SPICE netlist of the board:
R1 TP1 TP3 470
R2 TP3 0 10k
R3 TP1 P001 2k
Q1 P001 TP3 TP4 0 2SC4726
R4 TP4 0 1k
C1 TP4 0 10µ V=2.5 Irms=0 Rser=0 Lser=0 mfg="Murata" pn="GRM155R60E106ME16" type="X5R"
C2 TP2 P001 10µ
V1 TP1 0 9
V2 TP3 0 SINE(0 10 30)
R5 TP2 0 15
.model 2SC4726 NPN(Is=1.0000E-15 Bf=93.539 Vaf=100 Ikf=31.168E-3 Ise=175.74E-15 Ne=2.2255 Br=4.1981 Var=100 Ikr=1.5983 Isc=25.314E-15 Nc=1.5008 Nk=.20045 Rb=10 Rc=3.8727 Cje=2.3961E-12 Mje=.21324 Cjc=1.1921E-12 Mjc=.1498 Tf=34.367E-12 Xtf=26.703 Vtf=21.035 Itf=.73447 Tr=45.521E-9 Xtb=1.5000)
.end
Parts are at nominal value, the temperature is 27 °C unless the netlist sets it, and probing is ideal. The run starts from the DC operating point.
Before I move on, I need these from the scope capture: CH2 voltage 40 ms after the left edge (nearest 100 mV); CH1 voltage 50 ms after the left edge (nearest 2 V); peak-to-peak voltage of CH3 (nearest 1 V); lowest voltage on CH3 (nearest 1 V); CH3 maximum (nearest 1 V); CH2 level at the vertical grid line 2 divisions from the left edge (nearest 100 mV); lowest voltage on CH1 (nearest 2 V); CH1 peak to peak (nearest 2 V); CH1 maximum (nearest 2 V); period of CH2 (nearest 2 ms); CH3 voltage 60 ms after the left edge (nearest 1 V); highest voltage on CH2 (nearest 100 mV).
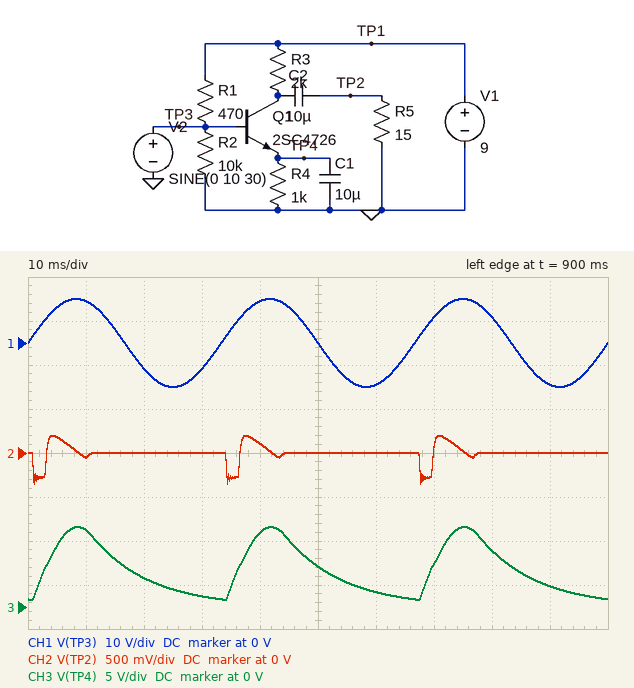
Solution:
100 mV
0 V
8 V
1 V
9 V
0 V
-10 V
20 V
10 V
34 ms
2 V
200 mV
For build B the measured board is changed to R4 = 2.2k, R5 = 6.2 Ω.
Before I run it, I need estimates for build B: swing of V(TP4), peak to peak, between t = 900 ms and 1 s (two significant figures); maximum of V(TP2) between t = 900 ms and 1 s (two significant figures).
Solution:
6.3 V
73 mV
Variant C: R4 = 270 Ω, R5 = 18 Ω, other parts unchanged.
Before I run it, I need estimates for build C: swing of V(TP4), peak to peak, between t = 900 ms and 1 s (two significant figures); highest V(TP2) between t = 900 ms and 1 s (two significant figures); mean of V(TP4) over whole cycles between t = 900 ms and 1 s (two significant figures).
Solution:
8.8 V
250 mV
2.9 V
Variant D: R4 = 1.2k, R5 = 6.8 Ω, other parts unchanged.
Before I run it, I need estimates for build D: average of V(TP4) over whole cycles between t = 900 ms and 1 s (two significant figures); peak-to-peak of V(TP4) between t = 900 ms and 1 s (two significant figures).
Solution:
4.6 V
7.9 V
